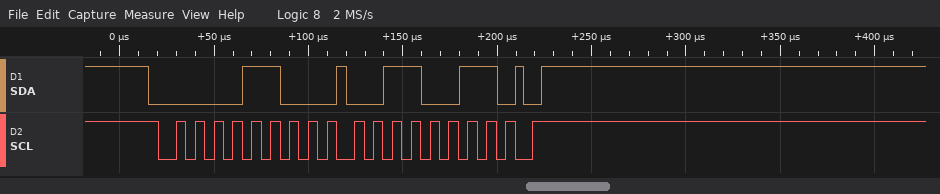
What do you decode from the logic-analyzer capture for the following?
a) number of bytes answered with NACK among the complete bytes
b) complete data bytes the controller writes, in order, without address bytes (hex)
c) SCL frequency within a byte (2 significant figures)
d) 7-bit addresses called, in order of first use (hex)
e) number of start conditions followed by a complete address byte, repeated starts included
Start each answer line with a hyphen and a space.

- 0
- 33
- 100 kHz
- 0x06
- 1
